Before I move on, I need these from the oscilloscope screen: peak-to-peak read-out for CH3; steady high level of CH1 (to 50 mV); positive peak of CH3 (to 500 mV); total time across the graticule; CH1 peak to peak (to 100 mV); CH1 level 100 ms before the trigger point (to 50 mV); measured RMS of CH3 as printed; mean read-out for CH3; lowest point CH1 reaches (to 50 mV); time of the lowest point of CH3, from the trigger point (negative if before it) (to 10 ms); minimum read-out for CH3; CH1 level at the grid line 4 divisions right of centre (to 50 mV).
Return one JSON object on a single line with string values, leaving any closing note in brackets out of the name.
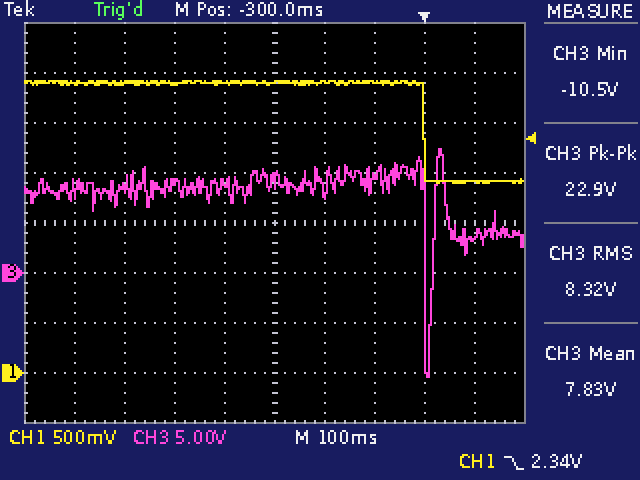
{"peak-to-peak read-out for CH3": "22.9 V", "steady high level of CH1": "2.90 V", "positive peak of CH3": "12.5 V", "total time across the graticule": "1 s", "CH1 peak to peak": "1.00 V", "CH1 level 100 ms before the trigger point": "2.90 V", "measured RMS of CH3 as printed": "8.32 V", "mean read-out for CH3": "7.83 V", "lowest point CH1 reaches": "1.90 V", "time of the lowest point of CH3, from the trigger point (negative if before it)": "+10 ms", "minimum read-out for CH3": "-10.5 V", "CH1 level at the grid line 4 divisions right of centre": "1.90 V"}
